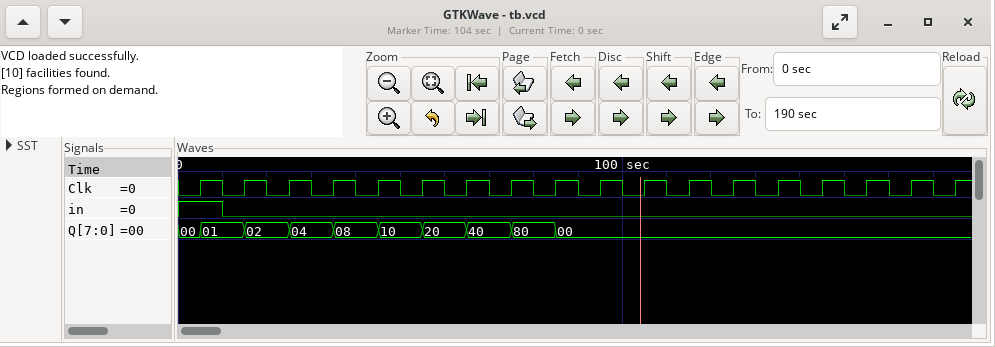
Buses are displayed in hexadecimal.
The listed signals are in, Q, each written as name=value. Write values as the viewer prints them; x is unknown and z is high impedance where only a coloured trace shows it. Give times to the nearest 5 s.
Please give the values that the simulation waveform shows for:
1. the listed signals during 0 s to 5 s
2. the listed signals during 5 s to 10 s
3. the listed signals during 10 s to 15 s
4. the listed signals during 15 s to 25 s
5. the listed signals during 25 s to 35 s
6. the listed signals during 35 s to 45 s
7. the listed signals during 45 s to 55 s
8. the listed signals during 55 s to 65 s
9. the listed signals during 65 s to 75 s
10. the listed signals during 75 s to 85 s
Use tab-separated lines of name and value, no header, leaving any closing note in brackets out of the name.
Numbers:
the listed signals during 0 s to 5 s	in=1, Q=00
the listed signals during 5 s to 10 s	in=1, Q=01
the listed signals during 10 s to 15 s	in=0, Q=01
the listed signals during 15 s to 25 s	in=0, Q=02
the listed signals during 25 s to 35 s	in=0, Q=04
the listed signals during 35 s to 45 s	in=0, Q=08
the listed signals during 45 s to 55 s	in=0, Q=10
the listed signals during 55 s to 65 s	in=0, Q=20
the listed signals during 65 s to 75 s	in=0, Q=40
the listed signals during 75 s to 85 s	in=0, Q=80
